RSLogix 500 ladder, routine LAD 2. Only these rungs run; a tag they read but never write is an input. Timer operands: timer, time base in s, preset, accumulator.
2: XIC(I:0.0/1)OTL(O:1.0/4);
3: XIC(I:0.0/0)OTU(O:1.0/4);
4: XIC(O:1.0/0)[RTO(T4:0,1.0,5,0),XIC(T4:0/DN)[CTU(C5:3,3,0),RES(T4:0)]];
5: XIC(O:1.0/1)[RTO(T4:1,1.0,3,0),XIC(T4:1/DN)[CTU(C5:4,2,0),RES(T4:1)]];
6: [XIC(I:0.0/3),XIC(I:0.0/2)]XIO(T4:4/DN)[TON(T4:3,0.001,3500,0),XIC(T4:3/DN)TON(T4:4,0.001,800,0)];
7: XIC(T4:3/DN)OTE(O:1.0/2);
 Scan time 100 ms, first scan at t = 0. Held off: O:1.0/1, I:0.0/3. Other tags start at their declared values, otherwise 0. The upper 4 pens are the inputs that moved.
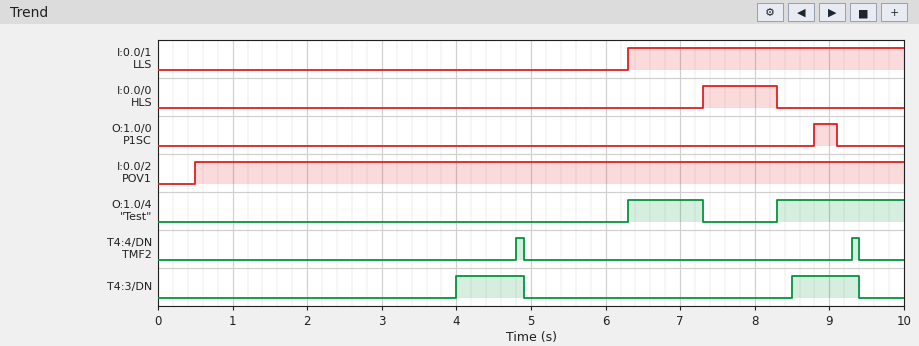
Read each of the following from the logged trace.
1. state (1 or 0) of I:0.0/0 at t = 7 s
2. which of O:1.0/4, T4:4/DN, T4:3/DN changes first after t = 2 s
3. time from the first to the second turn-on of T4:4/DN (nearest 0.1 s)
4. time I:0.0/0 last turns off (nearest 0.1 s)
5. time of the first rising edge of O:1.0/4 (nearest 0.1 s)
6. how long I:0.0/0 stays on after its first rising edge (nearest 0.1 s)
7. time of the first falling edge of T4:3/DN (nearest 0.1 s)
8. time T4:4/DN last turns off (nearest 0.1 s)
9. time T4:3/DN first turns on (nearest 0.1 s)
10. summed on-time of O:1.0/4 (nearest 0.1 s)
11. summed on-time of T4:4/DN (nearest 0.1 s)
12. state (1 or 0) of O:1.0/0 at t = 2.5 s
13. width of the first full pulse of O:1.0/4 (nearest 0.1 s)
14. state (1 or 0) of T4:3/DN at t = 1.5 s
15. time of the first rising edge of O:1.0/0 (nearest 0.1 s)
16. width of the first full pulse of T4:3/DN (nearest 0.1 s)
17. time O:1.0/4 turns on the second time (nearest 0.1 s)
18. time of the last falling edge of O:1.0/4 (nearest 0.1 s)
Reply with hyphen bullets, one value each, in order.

- 0
- T4:3/DN
- 4.5 s
- 8.3 s
- 6.3 s
- 1.0 s
- 4.9 s
- 9.4 s
- 4.0 s
- 2.7 s
- 0.2 s
- 0
- 1.0 s
- 0
- 8.8 s
- 0.9 s
- 8.3 s
- 7.3 s
